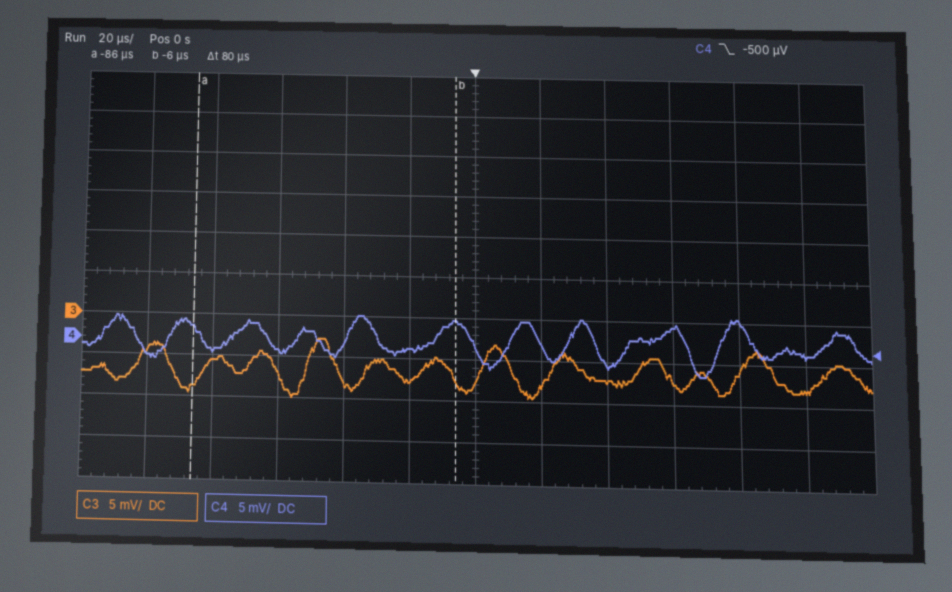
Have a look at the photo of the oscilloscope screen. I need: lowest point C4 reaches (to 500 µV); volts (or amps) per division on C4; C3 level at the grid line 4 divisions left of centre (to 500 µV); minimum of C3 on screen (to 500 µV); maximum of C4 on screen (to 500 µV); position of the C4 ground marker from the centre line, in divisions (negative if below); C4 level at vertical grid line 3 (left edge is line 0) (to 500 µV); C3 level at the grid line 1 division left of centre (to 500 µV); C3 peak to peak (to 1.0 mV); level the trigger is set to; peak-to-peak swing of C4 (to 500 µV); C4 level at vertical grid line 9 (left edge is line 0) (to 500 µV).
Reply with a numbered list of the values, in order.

1. -3.5 mV
2. 5 mV
3. -5.5 mV
4. -10.0 mV
5. 3.5 mV
6. -1.6 div
7. -1.5 mV
8. -7.5 mV
9. 7.0 mV
10. -500 µV
11. 7.0 mV
12. 2.5 mV
